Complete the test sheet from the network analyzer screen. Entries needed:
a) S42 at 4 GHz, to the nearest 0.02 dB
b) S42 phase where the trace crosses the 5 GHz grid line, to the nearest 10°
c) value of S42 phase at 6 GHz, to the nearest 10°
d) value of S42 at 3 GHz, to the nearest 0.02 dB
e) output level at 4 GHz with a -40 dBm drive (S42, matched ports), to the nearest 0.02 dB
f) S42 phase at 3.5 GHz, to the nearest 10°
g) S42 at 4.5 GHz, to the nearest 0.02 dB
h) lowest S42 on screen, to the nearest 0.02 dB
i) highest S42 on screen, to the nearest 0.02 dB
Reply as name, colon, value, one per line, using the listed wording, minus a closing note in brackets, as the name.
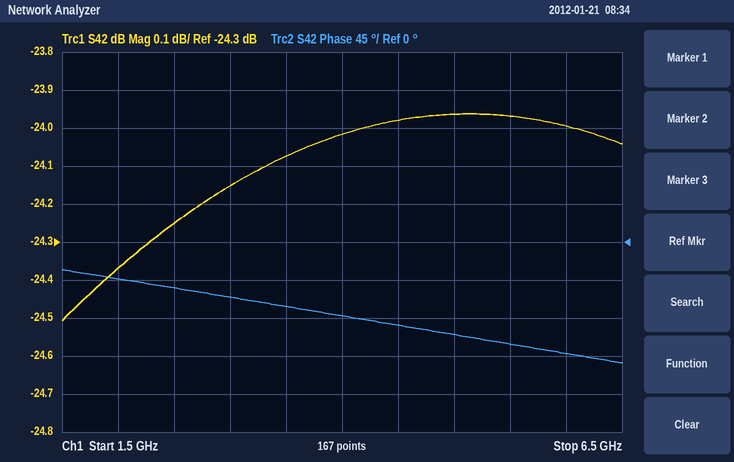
S42 at 4 GHz, to the nearest 0.02 dB: -24.02 dB
S42 phase where the trace crosses the 5 GHz grid line, to the nearest 10°: -110°
value of S42 phase at 6 GHz, to the nearest 10°: -130°
value of S42 at 3 GHz, to the nearest 0.02 dB: -24.16 dB
output level at 4 GHz with a -40 dBm drive (S42, matched ports), to the nearest 0.02 dB: -64.02 dBm
S42 phase at 3.5 GHz, to the nearest 10°: -80°
S42 at 4.5 GHz, to the nearest 0.02 dB: -23.98 dB
lowest S42 on screen, to the nearest 0.02 dB: -24.50 dB
highest S42 on screen, to the nearest 0.02 dB: -23.96 dB
